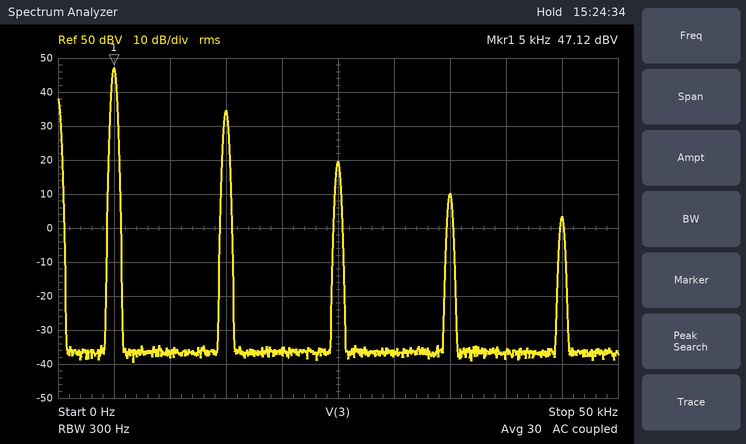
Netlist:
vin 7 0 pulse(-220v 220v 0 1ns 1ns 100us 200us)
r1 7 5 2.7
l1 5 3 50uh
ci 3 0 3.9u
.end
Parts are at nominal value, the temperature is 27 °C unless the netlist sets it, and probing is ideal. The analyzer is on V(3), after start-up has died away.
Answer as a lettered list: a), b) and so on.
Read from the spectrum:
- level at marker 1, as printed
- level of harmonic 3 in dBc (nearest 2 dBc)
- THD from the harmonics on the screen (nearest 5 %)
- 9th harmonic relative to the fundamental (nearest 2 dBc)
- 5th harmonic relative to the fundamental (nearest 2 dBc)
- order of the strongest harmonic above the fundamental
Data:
a) 47.12 dBV
b) -12 dBc
c) 25 %
d) -44 dBc
e) -28 dBc
f) 3
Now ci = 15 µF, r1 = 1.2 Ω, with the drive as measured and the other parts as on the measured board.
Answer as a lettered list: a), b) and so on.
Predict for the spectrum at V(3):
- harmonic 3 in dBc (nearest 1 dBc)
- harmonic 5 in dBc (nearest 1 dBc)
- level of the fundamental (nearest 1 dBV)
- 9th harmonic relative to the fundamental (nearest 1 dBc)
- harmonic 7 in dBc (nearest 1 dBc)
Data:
a) -29 dBc
b) -43 dBc
c) 50 dBV
d) -59 dBc
e) -52 dBc
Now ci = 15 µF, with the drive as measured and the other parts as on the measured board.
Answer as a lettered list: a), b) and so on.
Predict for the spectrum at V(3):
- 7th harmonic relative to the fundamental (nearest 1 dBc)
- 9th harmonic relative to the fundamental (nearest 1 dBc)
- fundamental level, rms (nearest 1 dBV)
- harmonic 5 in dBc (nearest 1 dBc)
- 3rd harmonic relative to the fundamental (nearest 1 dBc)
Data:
a) -46 dBc
b) -52 dBc
c) 44 dBV
d) -37 dBc
e) -24 dBc
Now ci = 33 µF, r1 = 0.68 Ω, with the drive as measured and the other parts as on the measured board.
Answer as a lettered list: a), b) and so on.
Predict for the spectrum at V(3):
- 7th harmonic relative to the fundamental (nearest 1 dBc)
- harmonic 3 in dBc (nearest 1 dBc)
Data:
a) -55 dBc
b) -33 dBc
